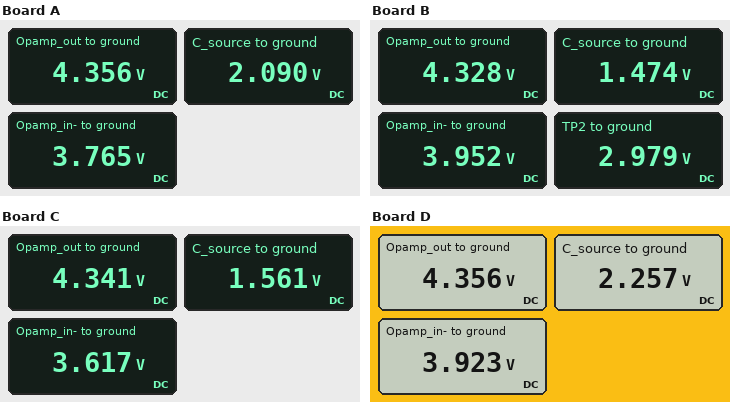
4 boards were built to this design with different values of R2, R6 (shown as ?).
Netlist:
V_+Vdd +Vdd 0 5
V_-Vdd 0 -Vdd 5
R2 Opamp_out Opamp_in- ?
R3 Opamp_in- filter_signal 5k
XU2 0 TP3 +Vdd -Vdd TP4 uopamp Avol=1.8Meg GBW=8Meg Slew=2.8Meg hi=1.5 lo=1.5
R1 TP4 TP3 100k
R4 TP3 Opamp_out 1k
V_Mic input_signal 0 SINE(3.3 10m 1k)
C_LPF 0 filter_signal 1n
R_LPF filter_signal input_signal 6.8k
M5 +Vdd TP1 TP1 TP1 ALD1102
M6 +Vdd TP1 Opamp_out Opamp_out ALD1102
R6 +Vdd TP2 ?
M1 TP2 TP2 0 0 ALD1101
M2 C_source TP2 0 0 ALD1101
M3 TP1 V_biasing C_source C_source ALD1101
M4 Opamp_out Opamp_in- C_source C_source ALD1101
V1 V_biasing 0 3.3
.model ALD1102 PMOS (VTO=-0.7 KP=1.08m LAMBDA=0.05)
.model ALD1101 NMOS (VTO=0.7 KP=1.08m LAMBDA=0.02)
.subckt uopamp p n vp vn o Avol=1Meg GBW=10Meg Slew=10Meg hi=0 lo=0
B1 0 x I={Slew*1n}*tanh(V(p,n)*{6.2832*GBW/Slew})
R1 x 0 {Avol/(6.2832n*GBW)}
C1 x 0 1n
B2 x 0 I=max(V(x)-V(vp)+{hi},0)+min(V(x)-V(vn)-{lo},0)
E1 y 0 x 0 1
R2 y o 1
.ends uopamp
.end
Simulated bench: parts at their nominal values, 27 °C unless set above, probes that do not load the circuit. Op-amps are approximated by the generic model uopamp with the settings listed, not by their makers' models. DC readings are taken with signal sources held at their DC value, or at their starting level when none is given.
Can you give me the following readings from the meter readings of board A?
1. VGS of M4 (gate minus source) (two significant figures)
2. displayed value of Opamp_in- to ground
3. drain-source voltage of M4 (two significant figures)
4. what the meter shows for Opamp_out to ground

1.7 V
3.765 V
2.3 V
4.356 V
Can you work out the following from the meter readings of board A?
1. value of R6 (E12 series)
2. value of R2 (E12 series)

4.7 kΩ
15 kΩ
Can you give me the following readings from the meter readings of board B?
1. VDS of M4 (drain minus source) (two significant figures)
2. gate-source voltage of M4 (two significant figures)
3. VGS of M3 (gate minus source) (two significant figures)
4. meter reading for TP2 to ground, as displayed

2.9 V
2.5 V
1.8 V
2.979 V
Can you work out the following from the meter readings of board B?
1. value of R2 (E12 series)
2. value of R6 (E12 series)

6.8 kΩ
680 Ω
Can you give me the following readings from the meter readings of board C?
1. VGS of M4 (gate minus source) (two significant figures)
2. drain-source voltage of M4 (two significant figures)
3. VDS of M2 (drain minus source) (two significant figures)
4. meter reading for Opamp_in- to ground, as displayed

2.1 V
2.8 V
1.6 V
3.617 V
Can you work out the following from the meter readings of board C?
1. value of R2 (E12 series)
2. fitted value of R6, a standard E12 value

27 kΩ
1.5 kΩ
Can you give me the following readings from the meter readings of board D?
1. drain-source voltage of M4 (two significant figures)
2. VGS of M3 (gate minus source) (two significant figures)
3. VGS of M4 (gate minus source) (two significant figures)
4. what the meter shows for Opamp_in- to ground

2.1 V
1.0 V
1.7 V
3.923 V
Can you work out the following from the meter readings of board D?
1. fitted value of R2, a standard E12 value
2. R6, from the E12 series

8.2 kΩ
5.6 kΩ
